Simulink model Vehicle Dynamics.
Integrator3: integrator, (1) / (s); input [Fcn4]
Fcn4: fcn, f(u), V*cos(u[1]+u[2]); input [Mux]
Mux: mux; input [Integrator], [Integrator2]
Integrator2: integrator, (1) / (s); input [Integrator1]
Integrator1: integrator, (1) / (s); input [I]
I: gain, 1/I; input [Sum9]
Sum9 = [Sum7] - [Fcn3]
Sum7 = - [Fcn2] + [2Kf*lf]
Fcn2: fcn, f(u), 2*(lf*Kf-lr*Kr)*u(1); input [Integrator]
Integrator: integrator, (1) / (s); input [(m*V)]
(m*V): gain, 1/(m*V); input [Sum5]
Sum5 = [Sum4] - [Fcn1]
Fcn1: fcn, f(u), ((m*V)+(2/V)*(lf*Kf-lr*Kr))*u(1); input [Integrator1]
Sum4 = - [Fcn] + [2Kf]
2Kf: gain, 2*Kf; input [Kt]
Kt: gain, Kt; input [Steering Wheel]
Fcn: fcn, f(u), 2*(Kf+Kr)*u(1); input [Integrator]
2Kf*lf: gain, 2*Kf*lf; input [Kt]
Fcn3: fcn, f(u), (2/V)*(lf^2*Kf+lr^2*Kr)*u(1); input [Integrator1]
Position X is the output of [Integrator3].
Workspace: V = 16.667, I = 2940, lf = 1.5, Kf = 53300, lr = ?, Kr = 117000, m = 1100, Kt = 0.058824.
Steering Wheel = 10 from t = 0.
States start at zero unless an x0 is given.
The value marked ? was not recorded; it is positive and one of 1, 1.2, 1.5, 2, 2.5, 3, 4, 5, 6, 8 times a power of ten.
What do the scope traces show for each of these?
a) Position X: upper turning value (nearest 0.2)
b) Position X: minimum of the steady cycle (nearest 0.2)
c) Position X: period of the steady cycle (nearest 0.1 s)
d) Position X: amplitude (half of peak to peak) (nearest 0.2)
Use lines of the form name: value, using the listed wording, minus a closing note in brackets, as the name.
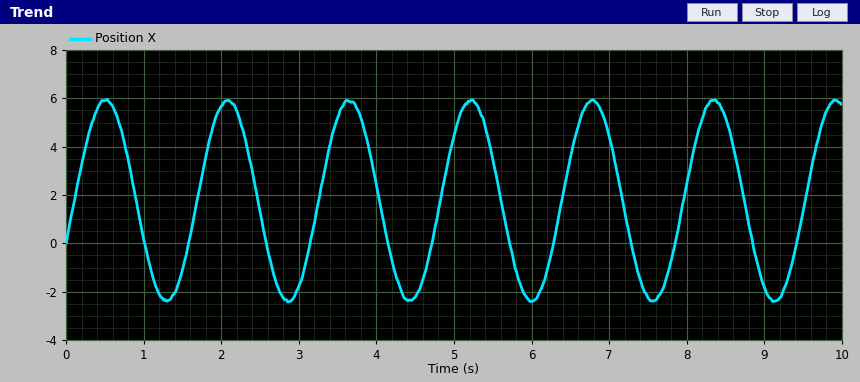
Position X: upper turning value: 6.0
Position X: minimum of the steady cycle: -2.4
Position X: period of the steady cycle: 1.6 s
Position X: amplitude (half of peak to peak): 4.2
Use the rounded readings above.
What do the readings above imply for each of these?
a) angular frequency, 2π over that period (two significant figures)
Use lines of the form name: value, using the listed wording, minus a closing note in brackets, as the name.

angular frequency, 2π over that period: 3.9 rad/s
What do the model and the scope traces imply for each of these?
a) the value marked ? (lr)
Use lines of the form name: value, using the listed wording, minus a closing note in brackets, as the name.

the value marked ?: 0.8
